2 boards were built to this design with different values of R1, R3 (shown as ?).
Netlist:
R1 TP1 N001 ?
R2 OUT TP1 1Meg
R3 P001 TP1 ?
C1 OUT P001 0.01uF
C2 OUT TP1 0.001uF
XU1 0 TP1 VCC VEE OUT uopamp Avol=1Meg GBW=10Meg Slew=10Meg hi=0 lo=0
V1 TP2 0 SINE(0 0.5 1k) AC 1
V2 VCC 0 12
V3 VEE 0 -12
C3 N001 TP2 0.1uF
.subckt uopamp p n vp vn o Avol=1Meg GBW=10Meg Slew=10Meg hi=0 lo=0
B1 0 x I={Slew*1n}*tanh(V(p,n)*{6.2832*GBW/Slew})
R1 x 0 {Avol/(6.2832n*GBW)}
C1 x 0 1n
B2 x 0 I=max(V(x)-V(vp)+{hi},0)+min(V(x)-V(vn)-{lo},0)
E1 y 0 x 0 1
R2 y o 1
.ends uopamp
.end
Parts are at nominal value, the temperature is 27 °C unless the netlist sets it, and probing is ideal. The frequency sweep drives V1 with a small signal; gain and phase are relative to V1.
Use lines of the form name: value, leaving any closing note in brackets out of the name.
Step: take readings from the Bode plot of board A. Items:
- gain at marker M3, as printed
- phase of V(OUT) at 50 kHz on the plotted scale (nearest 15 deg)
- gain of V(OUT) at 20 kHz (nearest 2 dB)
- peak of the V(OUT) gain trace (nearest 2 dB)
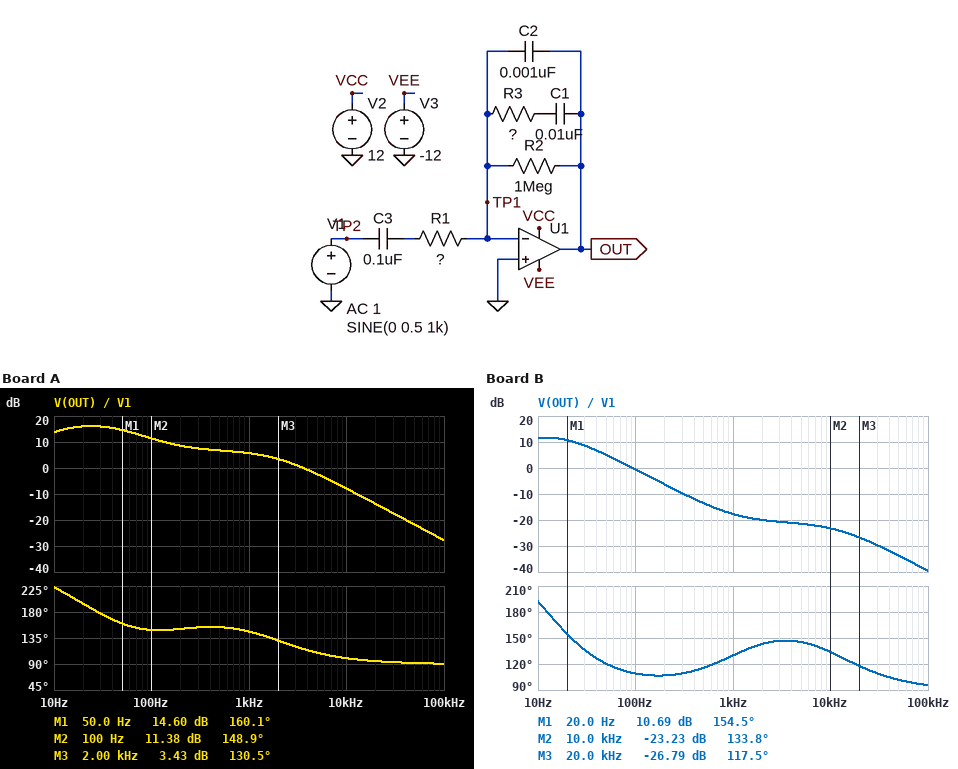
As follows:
gain at marker M3, as printed: 3.43 dB
phase of V(OUT) at 50 kHz on the plotted scale: 90 deg
gain of V(OUT) at 20 kHz: -14 dB
peak of the V(OUT) gain trace: 16 dB
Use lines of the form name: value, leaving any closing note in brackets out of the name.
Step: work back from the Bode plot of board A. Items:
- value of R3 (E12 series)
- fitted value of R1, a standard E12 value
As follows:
value of R3: 100 kΩ
fitted value of R1, a standard E12 value: 39 kΩ
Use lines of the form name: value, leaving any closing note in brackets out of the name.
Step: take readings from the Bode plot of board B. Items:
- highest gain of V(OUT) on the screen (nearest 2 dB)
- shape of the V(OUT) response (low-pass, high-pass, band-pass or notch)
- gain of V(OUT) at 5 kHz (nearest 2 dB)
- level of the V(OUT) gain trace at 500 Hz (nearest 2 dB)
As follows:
highest gain of V(OUT) on the screen: 12 dB
shape of the V(OUT) response: low-pass
gain of V(OUT) at 5 kHz: -22 dB
level of the V(OUT) gain trace at 500 Hz: -14 dB
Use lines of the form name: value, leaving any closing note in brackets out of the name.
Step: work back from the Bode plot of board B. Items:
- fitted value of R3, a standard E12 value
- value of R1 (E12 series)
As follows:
fitted value of R3, a standard E12 value: 15 kΩ
value of R1: 150 kΩ
